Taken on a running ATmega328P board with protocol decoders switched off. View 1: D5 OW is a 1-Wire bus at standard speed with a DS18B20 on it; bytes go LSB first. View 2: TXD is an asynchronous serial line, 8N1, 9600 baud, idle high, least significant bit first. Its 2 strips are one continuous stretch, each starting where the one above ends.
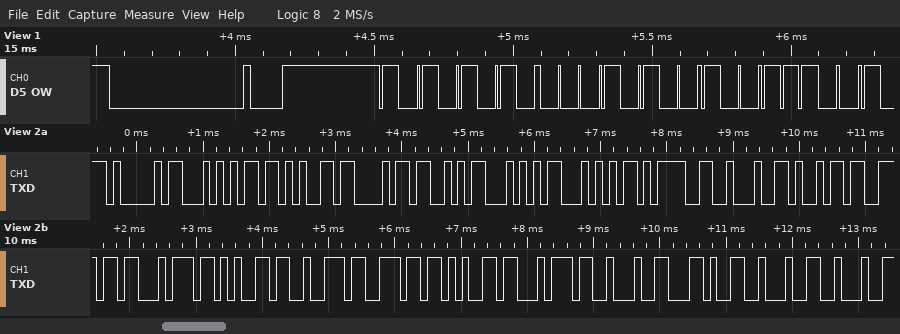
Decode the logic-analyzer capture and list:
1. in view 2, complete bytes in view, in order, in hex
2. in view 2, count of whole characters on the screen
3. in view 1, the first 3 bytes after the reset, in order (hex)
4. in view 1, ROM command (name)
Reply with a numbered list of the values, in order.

1. 41 54 2B 43 53 54 54 3D 22 69 6E 74 65 72 6E 65 74 22 2C 22 22
2. 21
3. 55 28 39
4. Match ROM
